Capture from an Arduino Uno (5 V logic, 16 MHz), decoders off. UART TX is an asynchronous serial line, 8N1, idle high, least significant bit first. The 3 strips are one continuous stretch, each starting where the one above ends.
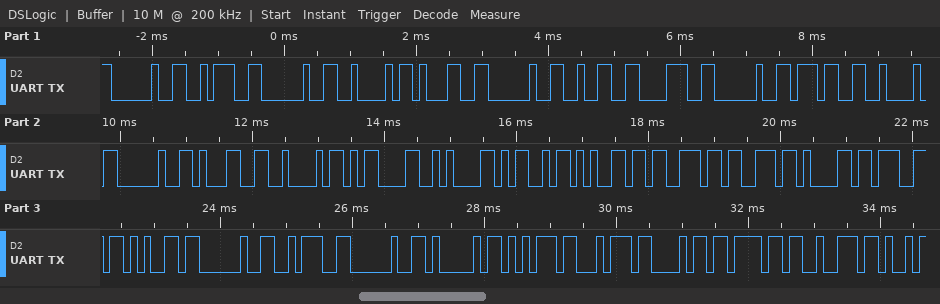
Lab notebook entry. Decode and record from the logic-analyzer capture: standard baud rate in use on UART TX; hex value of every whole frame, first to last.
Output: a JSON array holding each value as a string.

["9600 baud", "0x20 0x3A 0x20 0x42 0x31 0x20 0x32 0x38 0x20 0x37 0x42 0x20 0x31 0x42 0x0D 0x0A 0x4D 0x65 0x73 0x73 0x61 0x67 0x65 0x20 0x3A 0x20 0x41 0x75 0x74 0x68 0x6F 0x72"]
